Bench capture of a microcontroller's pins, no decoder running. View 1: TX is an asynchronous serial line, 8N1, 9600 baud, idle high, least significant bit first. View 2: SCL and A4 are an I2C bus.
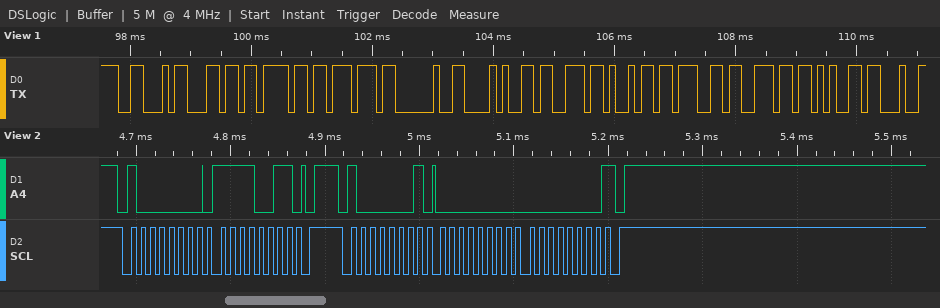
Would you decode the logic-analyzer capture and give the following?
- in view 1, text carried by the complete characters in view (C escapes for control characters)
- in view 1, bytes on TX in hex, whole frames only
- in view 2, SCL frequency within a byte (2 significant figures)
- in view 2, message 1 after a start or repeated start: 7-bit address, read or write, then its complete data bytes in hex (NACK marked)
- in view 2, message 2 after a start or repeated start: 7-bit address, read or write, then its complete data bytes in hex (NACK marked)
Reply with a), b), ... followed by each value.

a) "Flow (signe"
b) 46 6C 6F 77 20 28 73 69 67 6E 65
c) 100 kHz
d) 0x40 write: F3
e) 0x40 read: 00 00 NACK
